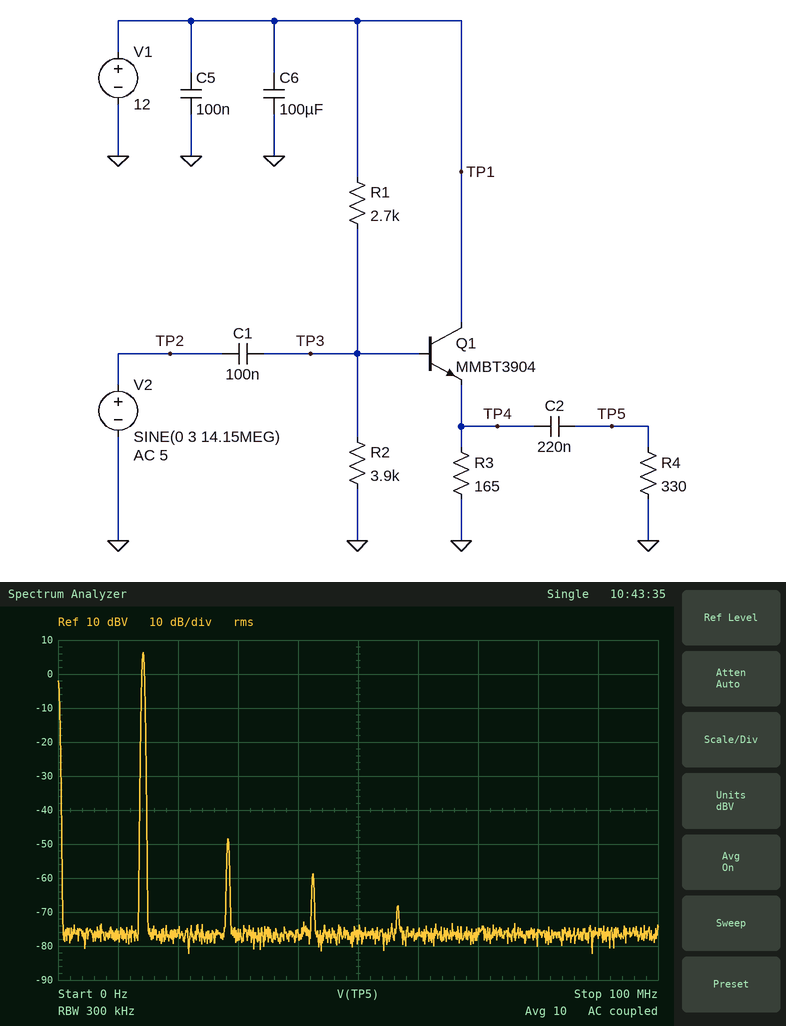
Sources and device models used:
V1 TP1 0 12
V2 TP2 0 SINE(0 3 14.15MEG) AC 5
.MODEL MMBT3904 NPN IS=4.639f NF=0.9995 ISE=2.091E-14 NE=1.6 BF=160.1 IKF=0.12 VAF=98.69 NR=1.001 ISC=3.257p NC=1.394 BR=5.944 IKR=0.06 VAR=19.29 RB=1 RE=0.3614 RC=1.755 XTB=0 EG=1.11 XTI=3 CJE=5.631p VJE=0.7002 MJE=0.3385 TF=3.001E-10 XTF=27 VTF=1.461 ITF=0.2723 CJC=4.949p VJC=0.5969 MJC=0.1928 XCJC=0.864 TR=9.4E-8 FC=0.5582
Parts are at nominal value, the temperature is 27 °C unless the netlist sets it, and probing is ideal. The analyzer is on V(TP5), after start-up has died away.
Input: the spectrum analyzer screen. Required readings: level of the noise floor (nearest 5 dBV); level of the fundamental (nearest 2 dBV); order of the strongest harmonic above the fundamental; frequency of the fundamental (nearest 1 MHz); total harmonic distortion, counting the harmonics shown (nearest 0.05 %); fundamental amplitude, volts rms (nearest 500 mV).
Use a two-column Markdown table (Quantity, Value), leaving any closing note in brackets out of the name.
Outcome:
| Quantity | Value |
|---|---|
| level of the noise floor | -75 dBV |
| level of the fundamental | 6 dBV |
| order of the strongest harmonic above the fundamental | 2 |
| frequency of the fundamental | 14 MHz |
| total harmonic distortion, counting the harmonics shown | 0.20 % |
| fundamental amplitude, volts rms | 2.0 V |
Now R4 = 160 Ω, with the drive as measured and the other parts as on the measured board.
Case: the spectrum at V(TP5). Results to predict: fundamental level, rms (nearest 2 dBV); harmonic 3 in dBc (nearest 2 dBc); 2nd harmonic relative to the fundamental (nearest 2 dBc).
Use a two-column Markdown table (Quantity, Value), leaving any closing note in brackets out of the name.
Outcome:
| Quantity | Value |
|---|---|
| fundamental level, rms | 6 dBV |
| harmonic 3 in dBc | -48 dBc |
| 2nd harmonic relative to the fundamental | -42 dBc |
